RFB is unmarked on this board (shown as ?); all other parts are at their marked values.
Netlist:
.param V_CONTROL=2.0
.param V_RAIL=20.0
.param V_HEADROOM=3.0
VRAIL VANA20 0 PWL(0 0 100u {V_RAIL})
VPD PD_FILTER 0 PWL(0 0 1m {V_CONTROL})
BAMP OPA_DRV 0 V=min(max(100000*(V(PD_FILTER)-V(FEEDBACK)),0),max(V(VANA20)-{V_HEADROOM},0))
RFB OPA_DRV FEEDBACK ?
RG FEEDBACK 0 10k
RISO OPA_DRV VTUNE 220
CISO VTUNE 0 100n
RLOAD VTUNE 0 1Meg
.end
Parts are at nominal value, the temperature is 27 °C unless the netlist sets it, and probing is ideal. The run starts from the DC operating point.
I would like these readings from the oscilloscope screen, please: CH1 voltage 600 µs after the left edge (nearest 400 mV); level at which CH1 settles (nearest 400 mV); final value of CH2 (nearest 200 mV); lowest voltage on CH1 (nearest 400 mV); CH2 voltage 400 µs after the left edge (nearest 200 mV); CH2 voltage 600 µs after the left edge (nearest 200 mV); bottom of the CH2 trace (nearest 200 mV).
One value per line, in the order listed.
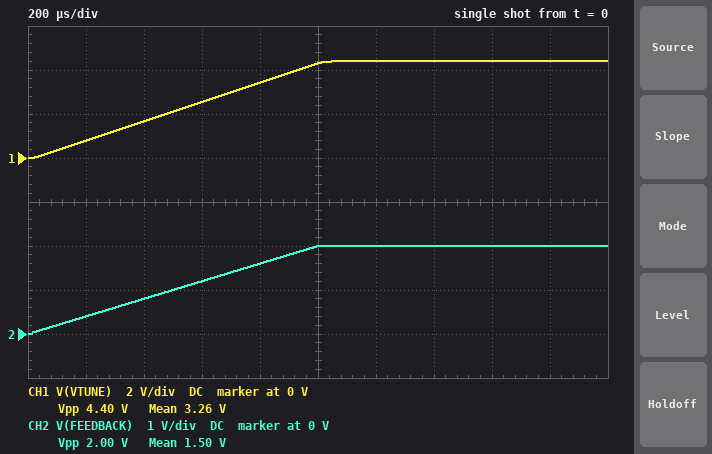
2.4 V
4.4 V
2.0 V
0 V
800 mV
1.2 V
0 V
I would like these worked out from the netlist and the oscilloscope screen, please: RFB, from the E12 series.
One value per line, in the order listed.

12 kΩ
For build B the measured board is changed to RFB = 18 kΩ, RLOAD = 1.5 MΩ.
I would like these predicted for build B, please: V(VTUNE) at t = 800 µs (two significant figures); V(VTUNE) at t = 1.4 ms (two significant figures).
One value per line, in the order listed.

4.4 V
5.6 V
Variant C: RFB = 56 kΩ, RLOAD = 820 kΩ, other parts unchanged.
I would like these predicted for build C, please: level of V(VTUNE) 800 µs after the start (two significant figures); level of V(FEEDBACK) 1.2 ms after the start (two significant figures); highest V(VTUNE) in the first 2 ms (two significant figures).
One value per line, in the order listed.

10 V
2.0 V
13 V
